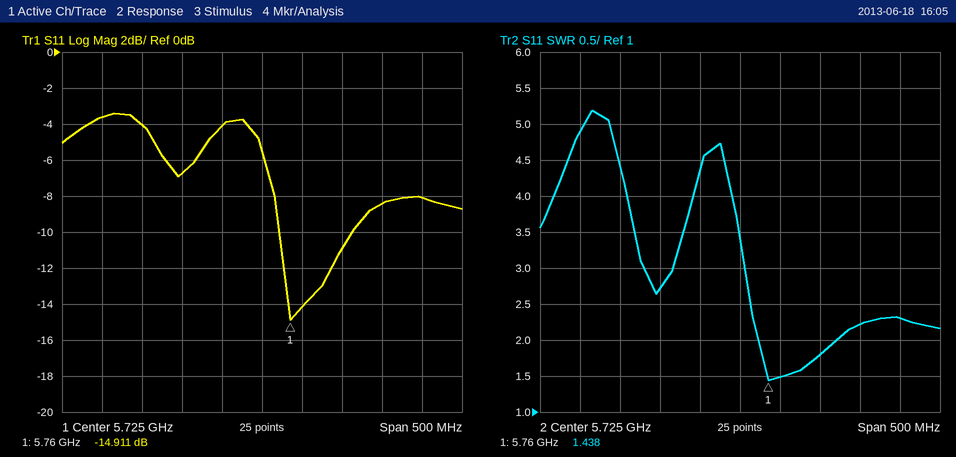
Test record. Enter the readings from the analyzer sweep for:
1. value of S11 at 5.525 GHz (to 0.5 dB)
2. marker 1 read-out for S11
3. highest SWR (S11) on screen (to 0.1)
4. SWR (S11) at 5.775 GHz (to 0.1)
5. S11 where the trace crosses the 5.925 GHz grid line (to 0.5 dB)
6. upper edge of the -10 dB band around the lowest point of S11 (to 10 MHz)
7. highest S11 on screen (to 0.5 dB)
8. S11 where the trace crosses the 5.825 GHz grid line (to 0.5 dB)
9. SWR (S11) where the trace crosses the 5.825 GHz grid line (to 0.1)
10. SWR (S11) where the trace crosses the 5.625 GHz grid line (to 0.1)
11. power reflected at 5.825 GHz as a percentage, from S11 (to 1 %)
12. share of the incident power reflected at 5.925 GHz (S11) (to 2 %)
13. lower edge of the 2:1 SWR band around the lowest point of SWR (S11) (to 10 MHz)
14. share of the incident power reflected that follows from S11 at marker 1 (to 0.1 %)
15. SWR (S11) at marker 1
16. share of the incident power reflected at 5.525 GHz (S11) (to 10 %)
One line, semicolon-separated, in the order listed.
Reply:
-3.5 dB; -14.911 dB; 5.2; 1.5; -8.0 dB; 5.84 GHz; -3.5 dB; -11.0 dB; 1.8; 2.7; 8 %; 16 %; 5.75 GHz; 3.2 %; 1.438; 40 %
